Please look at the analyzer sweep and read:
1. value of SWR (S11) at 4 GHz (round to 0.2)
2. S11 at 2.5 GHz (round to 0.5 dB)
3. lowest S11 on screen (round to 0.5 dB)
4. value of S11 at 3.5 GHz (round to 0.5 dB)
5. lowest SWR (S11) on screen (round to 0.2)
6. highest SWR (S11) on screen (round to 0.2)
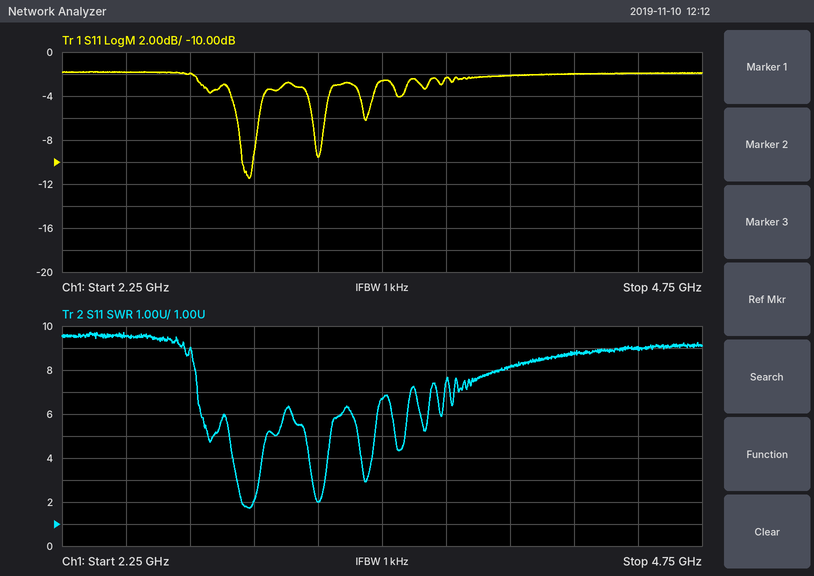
8.2
-2.0 dB
-11.5 dB
-2.5 dB
1.8
9.8
